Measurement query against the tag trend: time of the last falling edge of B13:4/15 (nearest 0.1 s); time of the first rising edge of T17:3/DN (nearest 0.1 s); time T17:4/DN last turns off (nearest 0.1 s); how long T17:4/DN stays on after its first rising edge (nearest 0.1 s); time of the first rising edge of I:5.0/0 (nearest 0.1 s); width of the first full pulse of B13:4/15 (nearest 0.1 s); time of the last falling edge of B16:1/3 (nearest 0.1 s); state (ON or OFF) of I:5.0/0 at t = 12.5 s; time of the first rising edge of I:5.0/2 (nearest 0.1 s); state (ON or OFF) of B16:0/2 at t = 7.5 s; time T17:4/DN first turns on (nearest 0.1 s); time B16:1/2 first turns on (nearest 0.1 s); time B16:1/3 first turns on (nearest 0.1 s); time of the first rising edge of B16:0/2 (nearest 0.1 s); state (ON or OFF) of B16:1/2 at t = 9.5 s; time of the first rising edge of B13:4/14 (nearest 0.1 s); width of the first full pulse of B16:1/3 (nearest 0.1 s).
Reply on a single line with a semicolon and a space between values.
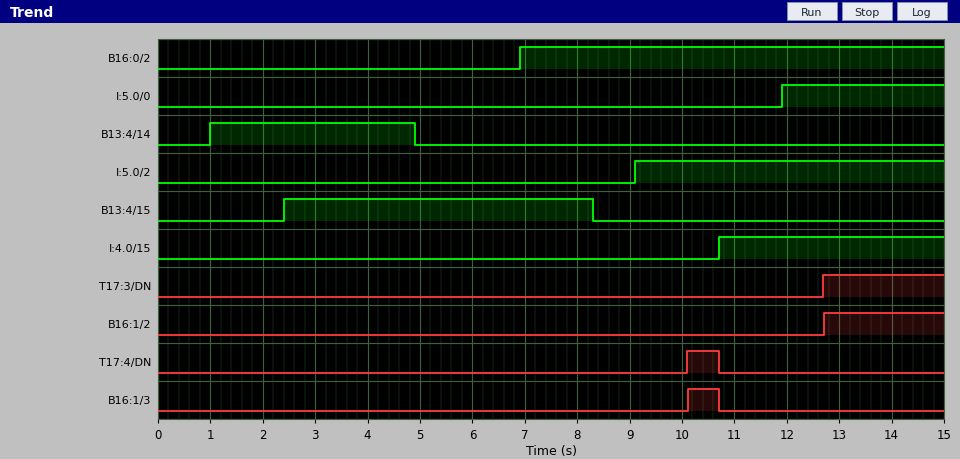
8.3 s; 12.7 s; 10.7 s; 0.6 s; 11.9 s; 5.9 s; 10.7 s; ON; 9.1 s; ON; 10.1 s; 12.7 s; 10.1 s; 6.9 s; OFF; 1.0 s; 0.6 s
